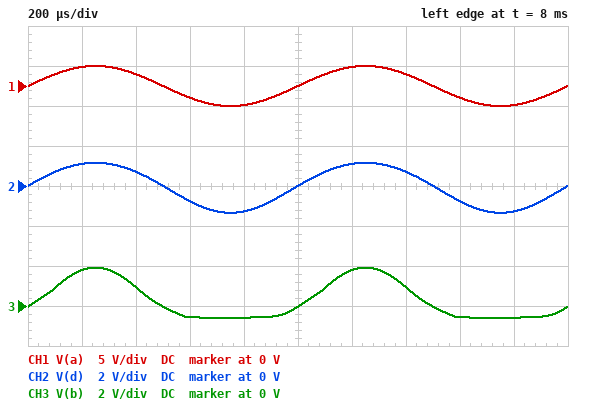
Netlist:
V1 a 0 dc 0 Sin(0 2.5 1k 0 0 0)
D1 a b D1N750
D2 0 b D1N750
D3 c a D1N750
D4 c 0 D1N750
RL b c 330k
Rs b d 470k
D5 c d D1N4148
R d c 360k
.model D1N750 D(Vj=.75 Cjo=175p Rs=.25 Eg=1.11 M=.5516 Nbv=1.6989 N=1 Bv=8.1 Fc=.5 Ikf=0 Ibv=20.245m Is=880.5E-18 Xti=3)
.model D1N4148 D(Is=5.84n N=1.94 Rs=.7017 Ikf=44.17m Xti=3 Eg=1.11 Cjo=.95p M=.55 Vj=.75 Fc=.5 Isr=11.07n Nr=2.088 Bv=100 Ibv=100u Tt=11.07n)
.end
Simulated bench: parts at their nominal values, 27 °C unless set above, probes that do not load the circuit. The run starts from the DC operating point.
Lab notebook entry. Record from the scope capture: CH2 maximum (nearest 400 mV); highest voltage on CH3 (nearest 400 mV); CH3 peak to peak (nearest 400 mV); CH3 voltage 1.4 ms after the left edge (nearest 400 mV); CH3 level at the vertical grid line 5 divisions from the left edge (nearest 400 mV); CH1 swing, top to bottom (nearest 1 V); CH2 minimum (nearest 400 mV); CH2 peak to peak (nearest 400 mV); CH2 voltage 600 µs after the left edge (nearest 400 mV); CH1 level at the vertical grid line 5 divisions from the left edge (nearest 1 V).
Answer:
1.2 V
2.0 V
2.4 V
800 mV
0 V
5 V
-1.2 V
2.4 V
-800 mV
0 V
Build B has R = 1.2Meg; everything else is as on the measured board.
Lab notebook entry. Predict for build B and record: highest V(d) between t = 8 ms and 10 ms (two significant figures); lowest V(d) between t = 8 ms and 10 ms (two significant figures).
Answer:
1.5 V
-960 mV
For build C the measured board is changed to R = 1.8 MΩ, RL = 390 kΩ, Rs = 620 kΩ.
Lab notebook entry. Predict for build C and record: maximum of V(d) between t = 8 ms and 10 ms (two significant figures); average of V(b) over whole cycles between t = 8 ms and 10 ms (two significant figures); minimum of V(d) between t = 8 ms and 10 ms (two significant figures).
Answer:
1.6 V
320 mV
-920 mV
